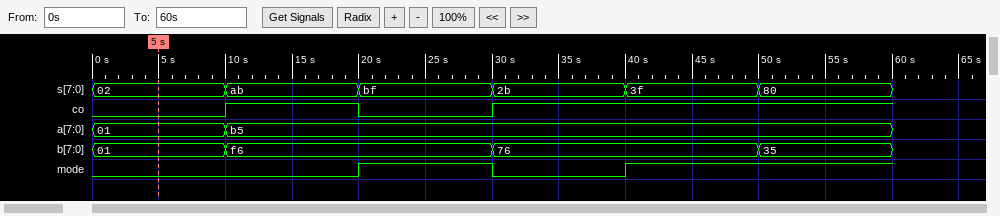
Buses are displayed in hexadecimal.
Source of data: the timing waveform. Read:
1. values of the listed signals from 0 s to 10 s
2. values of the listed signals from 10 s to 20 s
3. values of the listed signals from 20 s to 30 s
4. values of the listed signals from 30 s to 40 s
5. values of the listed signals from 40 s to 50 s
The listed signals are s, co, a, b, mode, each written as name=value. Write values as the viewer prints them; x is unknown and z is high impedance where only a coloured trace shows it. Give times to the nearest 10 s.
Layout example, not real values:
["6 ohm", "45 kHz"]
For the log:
["s=02, co=0, a=01, b=01, mode=0", "s=ab, co=1, a=b5, b=f6, mode=0", "s=bf, co=0, a=b5, b=f6, mode=1", "s=2b, co=1, a=b5, b=76, mode=0", "s=3f, co=1, a=b5, b=76, mode=1"]
